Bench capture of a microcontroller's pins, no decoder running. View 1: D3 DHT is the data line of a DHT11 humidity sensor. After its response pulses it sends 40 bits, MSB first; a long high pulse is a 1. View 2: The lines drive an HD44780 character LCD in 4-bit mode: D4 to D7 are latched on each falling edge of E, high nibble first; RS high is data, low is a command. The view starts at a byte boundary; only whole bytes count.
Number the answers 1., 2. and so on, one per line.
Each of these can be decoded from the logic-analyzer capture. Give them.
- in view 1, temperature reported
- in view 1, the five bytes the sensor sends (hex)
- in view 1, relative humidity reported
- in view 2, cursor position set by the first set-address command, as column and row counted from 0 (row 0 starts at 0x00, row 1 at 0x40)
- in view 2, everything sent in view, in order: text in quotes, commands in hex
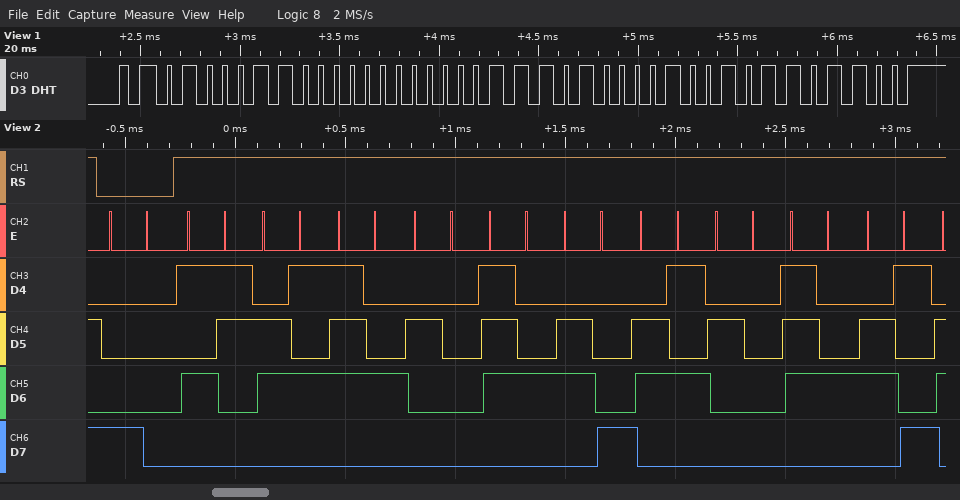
1. 29.9 °C
2. 46 00 1D 09 6C
3. 70 %
4. column 0, row 0
5. 0x80 "Set the ti"
